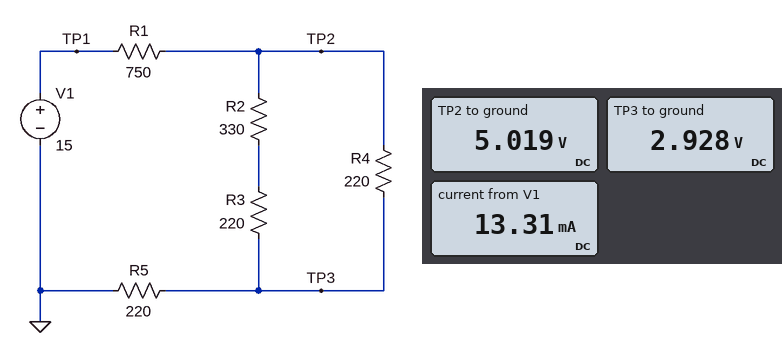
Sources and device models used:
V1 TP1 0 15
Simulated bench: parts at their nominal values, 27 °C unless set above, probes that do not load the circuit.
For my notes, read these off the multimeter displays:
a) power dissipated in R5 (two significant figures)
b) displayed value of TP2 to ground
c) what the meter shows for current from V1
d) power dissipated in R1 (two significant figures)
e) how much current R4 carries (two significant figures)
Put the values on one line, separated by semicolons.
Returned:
39 mW; 5.019 V; 13.31 mA; 130 mW; 9.5 mA
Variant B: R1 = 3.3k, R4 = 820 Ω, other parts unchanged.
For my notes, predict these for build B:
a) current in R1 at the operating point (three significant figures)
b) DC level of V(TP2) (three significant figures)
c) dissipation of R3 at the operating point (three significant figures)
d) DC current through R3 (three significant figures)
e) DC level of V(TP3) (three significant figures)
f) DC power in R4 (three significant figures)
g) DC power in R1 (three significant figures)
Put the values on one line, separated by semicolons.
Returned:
3.90 mA; 2.14 V; 1.20 mW; 2.33 mA; 857 mV; 2.01 mW; 50.1 mW
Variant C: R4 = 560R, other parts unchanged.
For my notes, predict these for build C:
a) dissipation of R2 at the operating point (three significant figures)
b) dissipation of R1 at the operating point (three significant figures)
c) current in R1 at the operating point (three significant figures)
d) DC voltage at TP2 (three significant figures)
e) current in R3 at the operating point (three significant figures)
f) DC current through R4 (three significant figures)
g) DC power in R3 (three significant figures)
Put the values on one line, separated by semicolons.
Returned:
12.1 mW; 108 mW; 12.0 mA; 5.98 V; 6.07 mA; 5.96 mA; 8.10 mW
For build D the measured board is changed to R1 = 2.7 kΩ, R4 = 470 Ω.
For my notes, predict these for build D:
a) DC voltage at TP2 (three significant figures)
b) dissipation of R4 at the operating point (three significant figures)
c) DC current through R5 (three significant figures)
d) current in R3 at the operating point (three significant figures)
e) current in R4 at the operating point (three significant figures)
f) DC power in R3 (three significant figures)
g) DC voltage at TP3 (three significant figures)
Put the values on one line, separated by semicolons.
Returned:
2.24 V; 3.05 mW; 4.73 mA; 2.18 mA; 2.55 mA; 1.04 mW; 1.04 V
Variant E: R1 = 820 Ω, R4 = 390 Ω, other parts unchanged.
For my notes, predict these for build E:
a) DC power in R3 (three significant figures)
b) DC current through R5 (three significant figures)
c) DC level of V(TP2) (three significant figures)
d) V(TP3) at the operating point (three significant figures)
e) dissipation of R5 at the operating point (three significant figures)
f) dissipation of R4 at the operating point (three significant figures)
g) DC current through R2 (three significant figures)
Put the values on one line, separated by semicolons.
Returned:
5.30 mW; 11.8 mA; 5.30 V; 2.60 V; 30.8 mW; 18.7 mW; 4.91 mA
